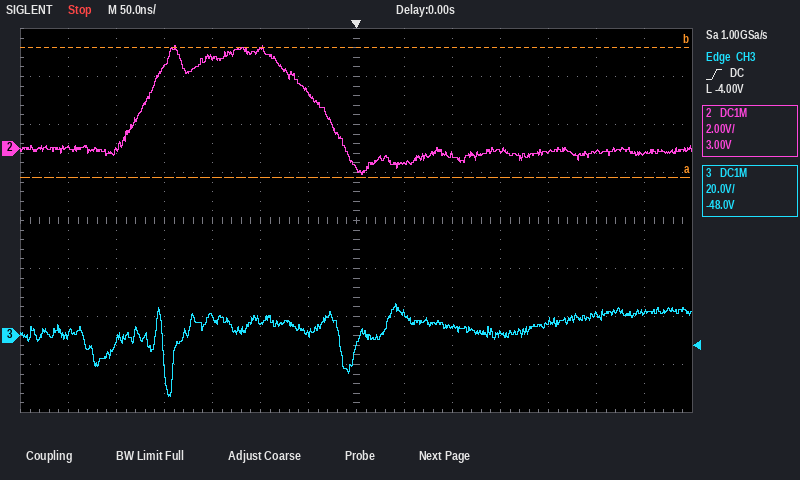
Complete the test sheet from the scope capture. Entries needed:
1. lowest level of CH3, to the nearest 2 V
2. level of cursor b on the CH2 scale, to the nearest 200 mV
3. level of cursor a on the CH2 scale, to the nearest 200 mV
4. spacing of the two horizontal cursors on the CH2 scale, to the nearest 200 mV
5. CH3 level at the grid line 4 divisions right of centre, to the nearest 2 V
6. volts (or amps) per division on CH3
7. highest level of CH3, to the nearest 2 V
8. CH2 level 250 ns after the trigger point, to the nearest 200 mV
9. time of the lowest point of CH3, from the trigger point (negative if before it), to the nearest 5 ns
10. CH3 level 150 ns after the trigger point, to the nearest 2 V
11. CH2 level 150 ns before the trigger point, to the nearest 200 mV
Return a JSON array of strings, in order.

["-26 V", "4.2 V", "-1.2 V", "5.4 V", "6 V", "20 V", "14 V", "-200 mV", "-195 ns", "0 V", "3.8 V"]
